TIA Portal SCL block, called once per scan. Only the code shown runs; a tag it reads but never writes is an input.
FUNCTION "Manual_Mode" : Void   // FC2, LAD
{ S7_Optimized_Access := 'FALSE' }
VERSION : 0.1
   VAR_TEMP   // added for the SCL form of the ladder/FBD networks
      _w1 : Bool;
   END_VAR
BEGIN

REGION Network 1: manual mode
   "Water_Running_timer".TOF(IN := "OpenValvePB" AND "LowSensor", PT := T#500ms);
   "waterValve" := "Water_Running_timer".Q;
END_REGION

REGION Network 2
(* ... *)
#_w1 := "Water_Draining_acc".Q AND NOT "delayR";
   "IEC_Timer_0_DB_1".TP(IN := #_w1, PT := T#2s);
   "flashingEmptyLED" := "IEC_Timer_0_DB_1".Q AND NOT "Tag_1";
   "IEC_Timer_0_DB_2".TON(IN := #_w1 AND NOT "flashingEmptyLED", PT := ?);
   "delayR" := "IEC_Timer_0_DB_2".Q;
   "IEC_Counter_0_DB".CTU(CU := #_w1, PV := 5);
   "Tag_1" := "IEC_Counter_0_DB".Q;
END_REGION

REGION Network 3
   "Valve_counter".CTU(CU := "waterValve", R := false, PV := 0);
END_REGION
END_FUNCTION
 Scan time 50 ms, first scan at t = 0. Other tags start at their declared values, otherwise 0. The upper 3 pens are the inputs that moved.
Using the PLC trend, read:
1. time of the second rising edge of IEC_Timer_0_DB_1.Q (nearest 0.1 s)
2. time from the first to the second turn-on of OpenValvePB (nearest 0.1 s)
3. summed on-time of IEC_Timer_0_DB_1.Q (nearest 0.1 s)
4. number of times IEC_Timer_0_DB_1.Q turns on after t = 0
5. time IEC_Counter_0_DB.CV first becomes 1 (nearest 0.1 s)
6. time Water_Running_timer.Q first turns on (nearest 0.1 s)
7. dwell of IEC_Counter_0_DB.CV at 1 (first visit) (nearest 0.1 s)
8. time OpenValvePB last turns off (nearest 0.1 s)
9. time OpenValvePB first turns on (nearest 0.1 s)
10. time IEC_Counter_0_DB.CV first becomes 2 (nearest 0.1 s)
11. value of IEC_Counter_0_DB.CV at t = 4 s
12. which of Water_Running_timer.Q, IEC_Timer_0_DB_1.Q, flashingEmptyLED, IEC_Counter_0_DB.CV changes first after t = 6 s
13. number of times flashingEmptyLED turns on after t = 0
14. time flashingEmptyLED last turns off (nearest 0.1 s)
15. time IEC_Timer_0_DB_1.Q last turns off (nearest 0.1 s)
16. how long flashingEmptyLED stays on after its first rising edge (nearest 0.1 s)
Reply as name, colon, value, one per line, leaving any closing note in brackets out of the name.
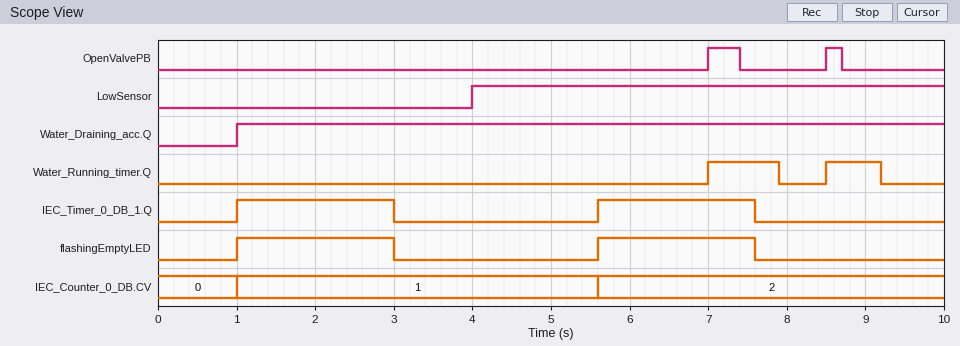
time of the second rising edge of IEC_Timer_0_DB_1.Q: 5.6 s
time from the first to the second turn-on of OpenValvePB: 1.5 s
summed on-time of IEC_Timer_0_DB_1.Q: 4.0 s
number of times IEC_Timer_0_DB_1.Q turns on after t = 0: 2
time IEC_Counter_0_DB.CV first becomes 1: 1.0 s
time Water_Running_timer.Q first turns on: 7.0 s
dwell of IEC_Counter_0_DB.CV at 1 (first visit): 4.6 s
time OpenValvePB last turns off: 8.7 s
time OpenValvePB first turns on: 7.0 s
time IEC_Counter_0_DB.CV first becomes 2: 5.6 s
value of IEC_Counter_0_DB.CV at t = 4 s: 1
which of Water_Running_timer.Q, IEC_Timer_0_DB_1.Q, flashingEmptyLED, IEC_Counter_0_DB.CV changes first after t = 6 s: Water_Running_timer.Q
number of times flashingEmptyLED turns on after t = 0: 2
time flashingEmptyLED last turns off: 7.6 s
time IEC_Timer_0_DB_1.Q last turns off: 7.6 s
how long flashingEmptyLED stays on after its first rising edge: 2.0 s
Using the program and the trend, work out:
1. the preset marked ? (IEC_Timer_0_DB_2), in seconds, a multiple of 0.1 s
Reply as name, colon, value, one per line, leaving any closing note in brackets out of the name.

the preset marked ? (IEC_Timer_0_DB_2), in seconds, a multiple of 0.1 s: 2.5 s
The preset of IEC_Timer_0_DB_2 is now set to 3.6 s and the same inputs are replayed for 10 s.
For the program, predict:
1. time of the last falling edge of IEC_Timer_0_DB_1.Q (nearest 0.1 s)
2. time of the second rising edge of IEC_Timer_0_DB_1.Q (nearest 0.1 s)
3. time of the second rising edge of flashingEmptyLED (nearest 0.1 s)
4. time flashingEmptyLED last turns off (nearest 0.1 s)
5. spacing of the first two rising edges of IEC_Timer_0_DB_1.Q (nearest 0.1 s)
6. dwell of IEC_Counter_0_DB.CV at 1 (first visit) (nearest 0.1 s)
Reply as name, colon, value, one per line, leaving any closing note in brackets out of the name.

time of the last falling edge of IEC_Timer_0_DB_1.Q: 8.7 s
time of the second rising edge of IEC_Timer_0_DB_1.Q: 6.7 s
time of the second rising edge of flashingEmptyLED: 6.7 s
time flashingEmptyLED last turns off: 8.7 s
spacing of the first two rising edges of IEC_Timer_0_DB_1.Q: 5.7 s
dwell of IEC_Counter_0_DB.CV at 1 (first visit): 5.7 s
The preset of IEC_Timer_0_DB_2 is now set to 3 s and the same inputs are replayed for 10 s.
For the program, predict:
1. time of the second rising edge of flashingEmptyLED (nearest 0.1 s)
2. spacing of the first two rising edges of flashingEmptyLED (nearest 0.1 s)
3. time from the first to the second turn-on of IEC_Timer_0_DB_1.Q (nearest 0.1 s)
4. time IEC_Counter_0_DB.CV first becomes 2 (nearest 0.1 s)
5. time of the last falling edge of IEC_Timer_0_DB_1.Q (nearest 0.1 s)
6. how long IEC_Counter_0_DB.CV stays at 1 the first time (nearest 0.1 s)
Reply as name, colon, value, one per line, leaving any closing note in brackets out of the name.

time of the second rising edge of flashingEmptyLED: 6.1 s
spacing of the first two rising edges of flashingEmptyLED: 5.1 s
time from the first to the second turn-on of IEC_Timer_0_DB_1.Q: 5.1 s
time IEC_Counter_0_DB.CV first becomes 2: 6.1 s
time of the last falling edge of IEC_Timer_0_DB_1.Q: 8.1 s
how long IEC_Counter_0_DB.CV stays at 1 the first time: 5.1 s
